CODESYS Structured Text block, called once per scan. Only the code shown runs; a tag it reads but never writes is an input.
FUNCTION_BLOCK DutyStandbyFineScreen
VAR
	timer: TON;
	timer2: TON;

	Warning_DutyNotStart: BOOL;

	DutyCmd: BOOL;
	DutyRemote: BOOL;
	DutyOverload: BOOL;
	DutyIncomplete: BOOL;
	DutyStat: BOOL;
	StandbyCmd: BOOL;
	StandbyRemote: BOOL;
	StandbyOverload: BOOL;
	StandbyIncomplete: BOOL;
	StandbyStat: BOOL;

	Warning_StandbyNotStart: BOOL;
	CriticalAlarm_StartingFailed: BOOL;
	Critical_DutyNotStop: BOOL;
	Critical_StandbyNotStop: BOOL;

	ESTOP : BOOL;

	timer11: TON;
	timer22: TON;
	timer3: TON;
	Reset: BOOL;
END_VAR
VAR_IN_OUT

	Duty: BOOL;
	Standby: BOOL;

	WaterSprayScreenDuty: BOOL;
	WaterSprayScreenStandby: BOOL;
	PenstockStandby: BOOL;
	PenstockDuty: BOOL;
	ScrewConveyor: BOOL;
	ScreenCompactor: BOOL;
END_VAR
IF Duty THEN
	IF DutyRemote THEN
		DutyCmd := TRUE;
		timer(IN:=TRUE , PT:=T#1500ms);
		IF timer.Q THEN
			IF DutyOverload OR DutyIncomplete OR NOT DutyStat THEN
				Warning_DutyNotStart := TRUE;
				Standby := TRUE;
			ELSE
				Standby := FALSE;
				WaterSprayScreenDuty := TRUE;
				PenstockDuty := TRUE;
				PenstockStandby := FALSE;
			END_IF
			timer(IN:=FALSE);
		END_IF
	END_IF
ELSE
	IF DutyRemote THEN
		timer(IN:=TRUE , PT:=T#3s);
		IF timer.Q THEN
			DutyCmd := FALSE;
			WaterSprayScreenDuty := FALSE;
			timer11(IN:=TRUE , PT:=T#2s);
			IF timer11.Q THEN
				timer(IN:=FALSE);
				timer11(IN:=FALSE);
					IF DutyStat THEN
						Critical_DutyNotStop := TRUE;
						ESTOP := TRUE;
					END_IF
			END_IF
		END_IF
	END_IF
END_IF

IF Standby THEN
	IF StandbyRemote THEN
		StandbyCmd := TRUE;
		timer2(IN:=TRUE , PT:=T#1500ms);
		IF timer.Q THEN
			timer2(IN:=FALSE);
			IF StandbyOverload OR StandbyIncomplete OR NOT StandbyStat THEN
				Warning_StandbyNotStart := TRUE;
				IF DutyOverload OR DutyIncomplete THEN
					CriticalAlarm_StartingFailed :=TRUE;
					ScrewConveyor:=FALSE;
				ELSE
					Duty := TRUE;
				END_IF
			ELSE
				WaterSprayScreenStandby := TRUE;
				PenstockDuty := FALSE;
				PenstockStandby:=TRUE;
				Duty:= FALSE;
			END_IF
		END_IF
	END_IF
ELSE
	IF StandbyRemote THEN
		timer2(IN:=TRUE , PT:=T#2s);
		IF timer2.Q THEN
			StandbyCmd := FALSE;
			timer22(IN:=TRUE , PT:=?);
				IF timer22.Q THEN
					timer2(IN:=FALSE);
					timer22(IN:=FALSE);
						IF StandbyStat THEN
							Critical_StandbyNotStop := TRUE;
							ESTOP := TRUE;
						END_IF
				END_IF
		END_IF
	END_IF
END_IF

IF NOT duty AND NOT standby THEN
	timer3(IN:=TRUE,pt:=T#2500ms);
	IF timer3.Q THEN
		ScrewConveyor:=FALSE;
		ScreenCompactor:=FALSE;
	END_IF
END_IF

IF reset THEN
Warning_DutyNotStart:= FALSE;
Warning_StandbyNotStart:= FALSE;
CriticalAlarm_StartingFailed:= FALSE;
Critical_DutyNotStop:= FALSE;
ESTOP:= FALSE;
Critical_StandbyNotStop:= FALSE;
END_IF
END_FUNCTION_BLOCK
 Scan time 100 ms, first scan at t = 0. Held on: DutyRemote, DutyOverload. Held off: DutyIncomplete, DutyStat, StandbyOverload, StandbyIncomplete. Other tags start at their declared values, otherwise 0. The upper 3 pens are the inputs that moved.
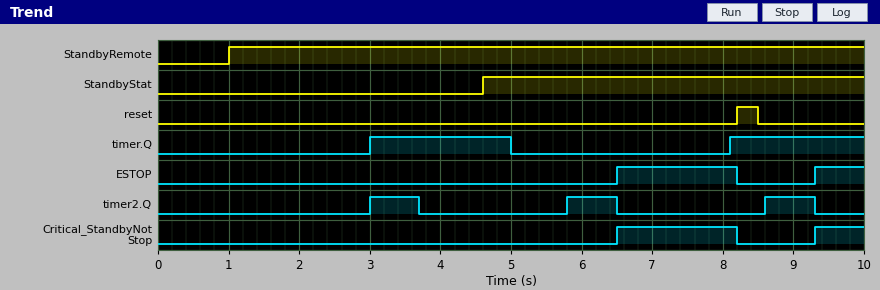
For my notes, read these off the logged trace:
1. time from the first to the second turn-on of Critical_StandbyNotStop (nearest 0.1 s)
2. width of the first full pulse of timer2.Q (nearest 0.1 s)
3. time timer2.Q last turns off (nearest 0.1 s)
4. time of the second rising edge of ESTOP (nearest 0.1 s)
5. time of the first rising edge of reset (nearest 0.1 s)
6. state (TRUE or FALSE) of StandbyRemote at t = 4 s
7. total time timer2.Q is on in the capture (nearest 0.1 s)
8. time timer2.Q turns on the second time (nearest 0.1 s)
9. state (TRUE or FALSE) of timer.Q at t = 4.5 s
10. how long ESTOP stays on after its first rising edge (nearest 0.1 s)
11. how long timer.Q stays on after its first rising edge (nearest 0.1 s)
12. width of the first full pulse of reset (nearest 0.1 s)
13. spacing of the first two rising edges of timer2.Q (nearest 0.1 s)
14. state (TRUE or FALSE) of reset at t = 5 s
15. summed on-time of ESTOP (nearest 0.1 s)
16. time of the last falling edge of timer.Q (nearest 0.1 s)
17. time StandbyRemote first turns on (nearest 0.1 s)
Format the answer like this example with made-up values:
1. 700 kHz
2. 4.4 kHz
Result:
1. 2.8 s
2. 0.7 s
3. 9.3 s
4. 9.3 s
5. 8.2 s
6. TRUE
7. 2.1 s
8. 5.8 s
9. TRUE
10. 1.7 s
11. 2.0 s
12. 0.3 s
13. 2.8 s
14. FALSE
15. 2.4 s
16. 5.0 s
17. 1.0 s
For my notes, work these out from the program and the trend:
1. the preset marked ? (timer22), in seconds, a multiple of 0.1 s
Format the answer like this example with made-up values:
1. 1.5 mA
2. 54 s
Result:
1. 0.7 s
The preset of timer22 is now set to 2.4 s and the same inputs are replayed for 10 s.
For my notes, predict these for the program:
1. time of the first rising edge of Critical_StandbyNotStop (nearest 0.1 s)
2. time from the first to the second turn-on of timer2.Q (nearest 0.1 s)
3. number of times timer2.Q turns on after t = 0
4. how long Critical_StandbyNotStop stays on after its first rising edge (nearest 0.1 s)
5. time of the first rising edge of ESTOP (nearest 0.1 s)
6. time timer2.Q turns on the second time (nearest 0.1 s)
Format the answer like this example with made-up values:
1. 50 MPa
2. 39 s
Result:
1. 5.4 s
2. 4.5 s
3. 2
4. 2.8 s
5. 5.4 s
6. 7.5 s
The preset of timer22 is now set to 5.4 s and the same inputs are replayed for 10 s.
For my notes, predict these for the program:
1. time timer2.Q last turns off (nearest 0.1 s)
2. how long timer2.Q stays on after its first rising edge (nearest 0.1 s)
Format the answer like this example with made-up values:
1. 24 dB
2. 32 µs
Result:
1. 8.4 s
2. 5.4 s
